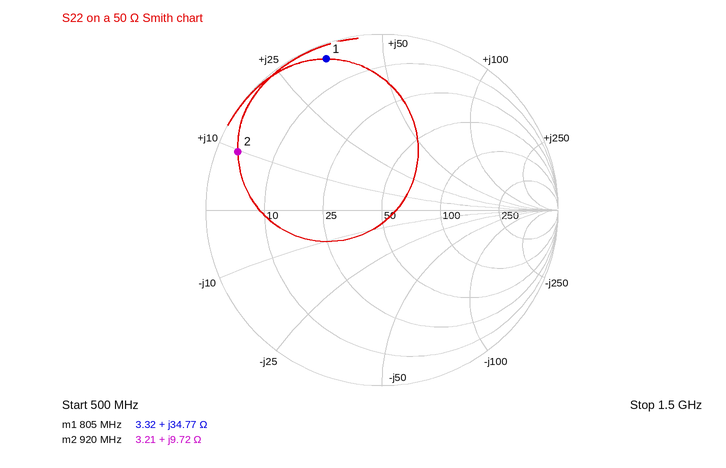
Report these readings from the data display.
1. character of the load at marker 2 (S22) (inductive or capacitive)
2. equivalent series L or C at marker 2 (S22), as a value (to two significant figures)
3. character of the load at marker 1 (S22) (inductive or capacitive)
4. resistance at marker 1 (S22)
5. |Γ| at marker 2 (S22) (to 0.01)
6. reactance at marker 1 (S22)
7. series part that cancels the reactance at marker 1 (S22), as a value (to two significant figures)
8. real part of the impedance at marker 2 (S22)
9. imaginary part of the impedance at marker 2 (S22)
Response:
inductive
1.7 nH
inductive
3.32 Ω
0.88
+34.77 Ω
5.7 pF
3.21 Ω
+9.72 Ω
